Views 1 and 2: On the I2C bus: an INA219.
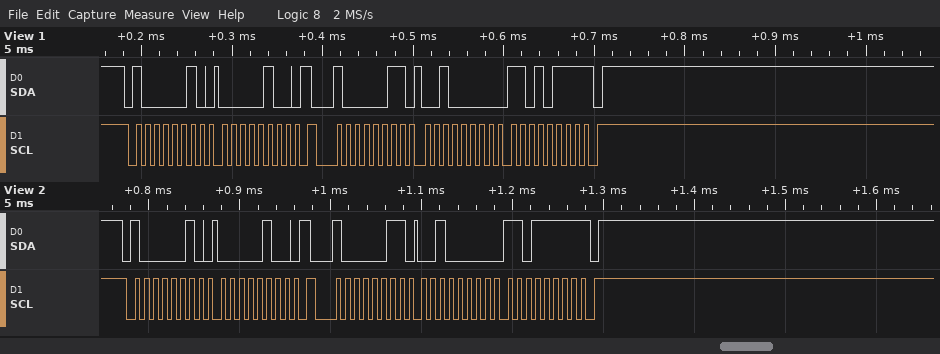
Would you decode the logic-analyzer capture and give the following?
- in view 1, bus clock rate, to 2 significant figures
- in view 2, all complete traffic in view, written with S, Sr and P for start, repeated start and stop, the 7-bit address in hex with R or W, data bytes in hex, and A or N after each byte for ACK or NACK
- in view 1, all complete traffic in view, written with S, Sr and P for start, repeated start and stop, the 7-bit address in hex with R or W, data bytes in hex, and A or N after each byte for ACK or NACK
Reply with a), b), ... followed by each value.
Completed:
a) 100 kHz
b) S 41W A 04 A Sr 41R A 20 A DF N P
c) S 41W A 04 A Sr 41R A 20 A D7 N P
